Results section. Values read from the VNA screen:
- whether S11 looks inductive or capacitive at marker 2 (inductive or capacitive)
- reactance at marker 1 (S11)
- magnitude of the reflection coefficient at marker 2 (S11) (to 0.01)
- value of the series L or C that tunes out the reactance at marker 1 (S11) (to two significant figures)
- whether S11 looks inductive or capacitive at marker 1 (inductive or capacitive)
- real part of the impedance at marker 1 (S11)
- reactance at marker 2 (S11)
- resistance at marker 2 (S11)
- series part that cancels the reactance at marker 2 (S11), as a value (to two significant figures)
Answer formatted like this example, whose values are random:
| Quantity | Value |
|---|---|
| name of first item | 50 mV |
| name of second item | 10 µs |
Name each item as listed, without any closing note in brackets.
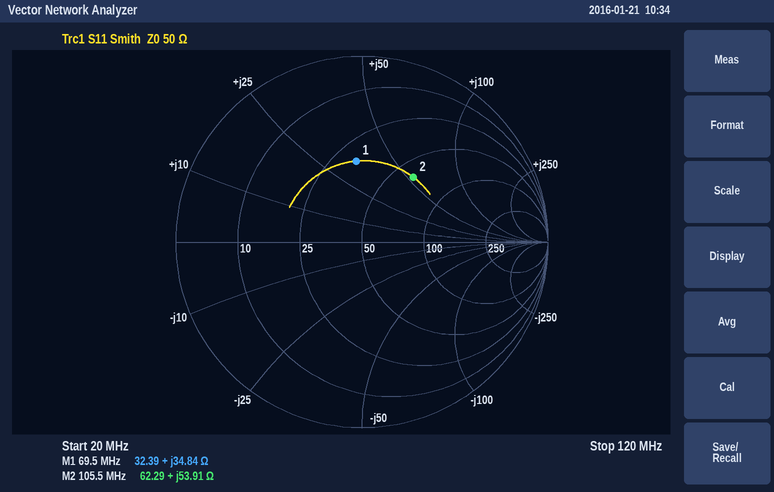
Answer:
| Quantity | Value |
|---|---|
| whether S11 looks inductive or capacitive at marker 2 | inductive |
| reactance at marker 1 | +34.84 Ω |
| magnitude of the reflection coefficient at marker 2 (S11) | 0.44 |
| value of the series L or C that tunes out the reactance at marker 1 (S11) | 66 pF |
| whether S11 looks inductive or capacitive at marker 1 | inductive |
| real part of the impedance at marker 1 | 32.39 Ω |
| reactance at marker 2 | +53.91 Ω |
| resistance at marker 2 | 62.29 Ω |
| series part that cancels the reactance at marker 2 (S11), as a value | 28 pF |
